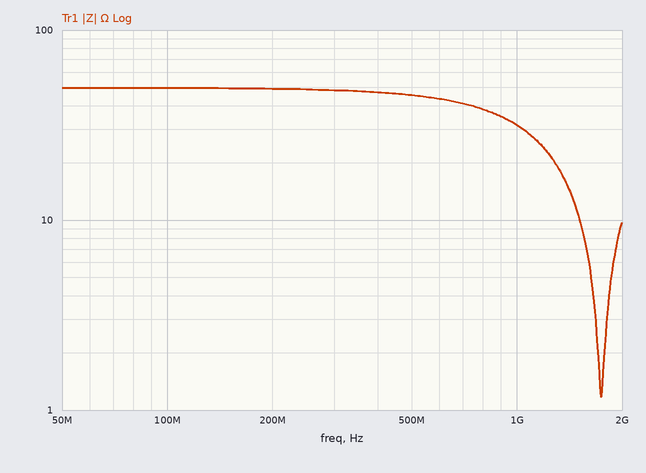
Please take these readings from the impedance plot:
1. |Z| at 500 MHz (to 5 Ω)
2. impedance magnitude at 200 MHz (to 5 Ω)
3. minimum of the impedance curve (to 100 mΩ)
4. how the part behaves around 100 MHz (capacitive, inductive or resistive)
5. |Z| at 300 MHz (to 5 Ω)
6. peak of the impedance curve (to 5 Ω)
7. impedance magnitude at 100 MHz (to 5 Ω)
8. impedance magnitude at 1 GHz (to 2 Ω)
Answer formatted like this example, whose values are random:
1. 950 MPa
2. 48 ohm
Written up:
1. 45 Ω
2. 50 Ω
3. 1.2 Ω
4. resistive
5. 50 Ω
6. 50 Ω
7. 50 Ω
8. 32 Ω
